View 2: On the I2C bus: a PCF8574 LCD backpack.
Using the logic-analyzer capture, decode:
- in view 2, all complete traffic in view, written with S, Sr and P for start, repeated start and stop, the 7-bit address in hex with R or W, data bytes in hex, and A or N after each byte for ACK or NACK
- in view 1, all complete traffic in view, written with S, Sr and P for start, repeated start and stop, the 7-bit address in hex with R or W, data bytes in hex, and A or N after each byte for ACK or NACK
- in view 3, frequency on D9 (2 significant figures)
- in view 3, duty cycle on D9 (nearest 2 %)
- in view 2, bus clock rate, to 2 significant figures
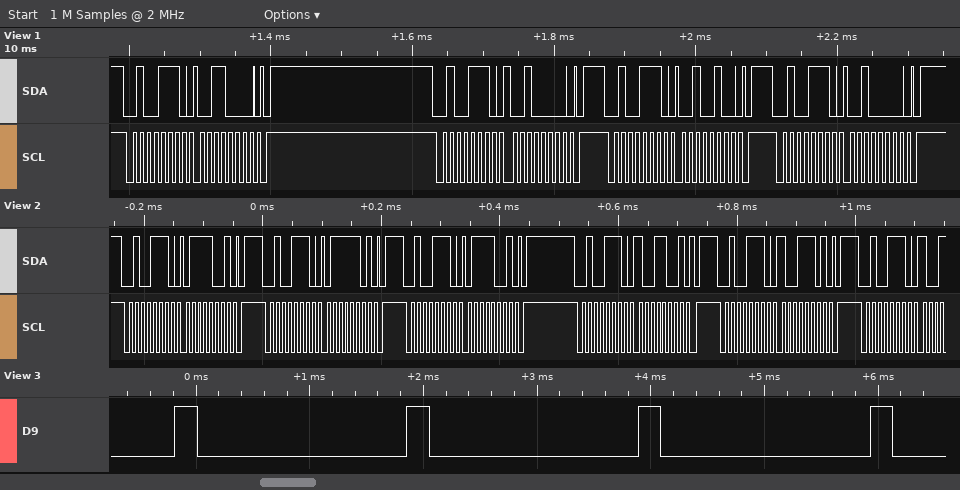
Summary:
S 27W A 79 A P S 27W A 7D A P S 27W A 79 A P S 27W A 99 A P S 27W A 9D A P S 27W A
S 27W A 30 A P S 27W A 20 A P S 27W A 24 A P S 27W A 20 A P
490 Hz
10 %
100 kHz
